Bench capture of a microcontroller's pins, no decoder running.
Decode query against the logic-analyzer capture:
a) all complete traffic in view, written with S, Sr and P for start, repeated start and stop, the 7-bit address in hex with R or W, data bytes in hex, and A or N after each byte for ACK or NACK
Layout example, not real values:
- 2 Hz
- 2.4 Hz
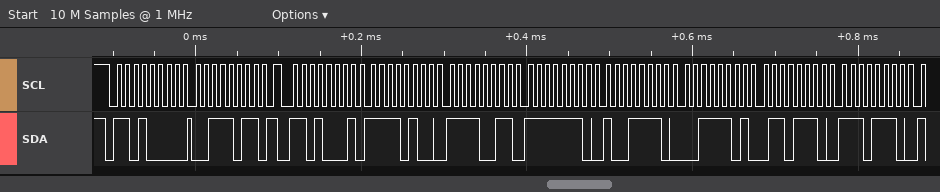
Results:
- S 68W A 3B A Sr 68R A F4 A F3 A FE A 9E A 3D A 6E A EE A
